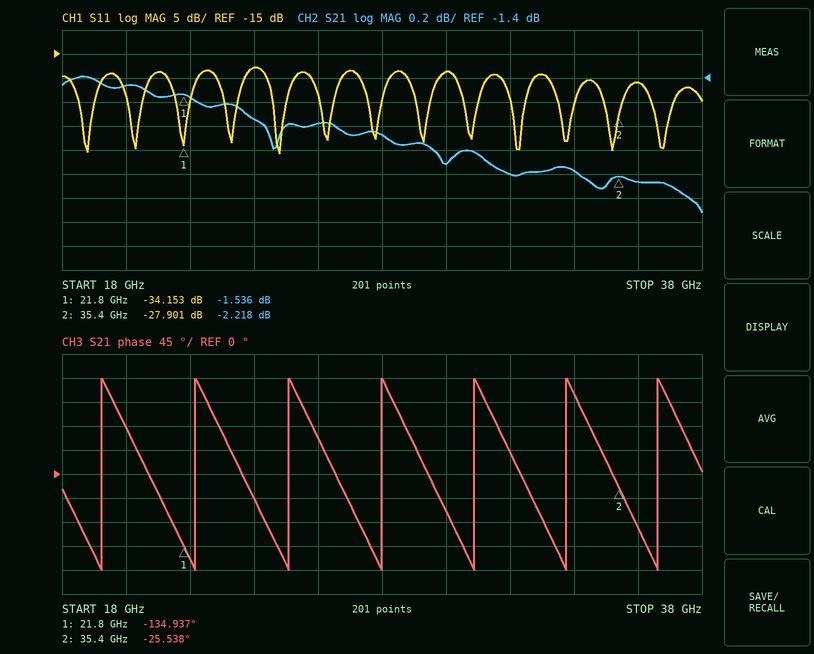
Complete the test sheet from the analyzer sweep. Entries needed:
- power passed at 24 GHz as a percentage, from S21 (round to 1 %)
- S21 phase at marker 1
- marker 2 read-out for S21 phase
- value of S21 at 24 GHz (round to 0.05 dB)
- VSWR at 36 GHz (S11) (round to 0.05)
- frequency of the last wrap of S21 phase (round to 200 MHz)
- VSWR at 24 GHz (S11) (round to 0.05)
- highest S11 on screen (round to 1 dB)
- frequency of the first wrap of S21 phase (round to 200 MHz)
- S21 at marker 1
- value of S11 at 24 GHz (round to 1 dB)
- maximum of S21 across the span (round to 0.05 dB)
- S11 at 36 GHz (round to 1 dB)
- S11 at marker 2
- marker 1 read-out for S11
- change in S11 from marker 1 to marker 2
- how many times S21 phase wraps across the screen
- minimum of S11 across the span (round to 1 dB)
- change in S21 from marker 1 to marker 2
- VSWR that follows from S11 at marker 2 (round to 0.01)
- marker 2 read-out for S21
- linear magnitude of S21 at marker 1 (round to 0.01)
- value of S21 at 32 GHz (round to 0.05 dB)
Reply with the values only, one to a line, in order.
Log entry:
67 %
-134.937°
-25.538°
-1.75 dB
1.20
36.6 GHz
1.30
-18 dB
19.2 GHz
-1.536 dB
-18 dB
-1.40 dB
-21 dB
-27.901 dB
-34.153 dB
6.252 dB
7
-36 dB
-0.682 dB
1.08
-2.218 dB
0.84
-2.20 dB
